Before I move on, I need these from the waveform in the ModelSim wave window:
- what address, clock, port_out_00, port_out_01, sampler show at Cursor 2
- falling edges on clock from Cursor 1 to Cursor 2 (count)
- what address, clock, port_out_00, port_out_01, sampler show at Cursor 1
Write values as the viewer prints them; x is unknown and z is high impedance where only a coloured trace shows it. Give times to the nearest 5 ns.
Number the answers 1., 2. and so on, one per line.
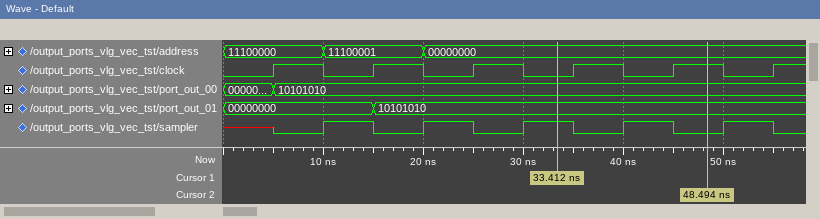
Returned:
1. address=00000000, clock=1, port_out_00=10101010, port_out_01=10101010, sampler=0
2. 1
3. address=00000000, clock=0, port_out_00=10101010, port_out_01=10101010, sampler=1
